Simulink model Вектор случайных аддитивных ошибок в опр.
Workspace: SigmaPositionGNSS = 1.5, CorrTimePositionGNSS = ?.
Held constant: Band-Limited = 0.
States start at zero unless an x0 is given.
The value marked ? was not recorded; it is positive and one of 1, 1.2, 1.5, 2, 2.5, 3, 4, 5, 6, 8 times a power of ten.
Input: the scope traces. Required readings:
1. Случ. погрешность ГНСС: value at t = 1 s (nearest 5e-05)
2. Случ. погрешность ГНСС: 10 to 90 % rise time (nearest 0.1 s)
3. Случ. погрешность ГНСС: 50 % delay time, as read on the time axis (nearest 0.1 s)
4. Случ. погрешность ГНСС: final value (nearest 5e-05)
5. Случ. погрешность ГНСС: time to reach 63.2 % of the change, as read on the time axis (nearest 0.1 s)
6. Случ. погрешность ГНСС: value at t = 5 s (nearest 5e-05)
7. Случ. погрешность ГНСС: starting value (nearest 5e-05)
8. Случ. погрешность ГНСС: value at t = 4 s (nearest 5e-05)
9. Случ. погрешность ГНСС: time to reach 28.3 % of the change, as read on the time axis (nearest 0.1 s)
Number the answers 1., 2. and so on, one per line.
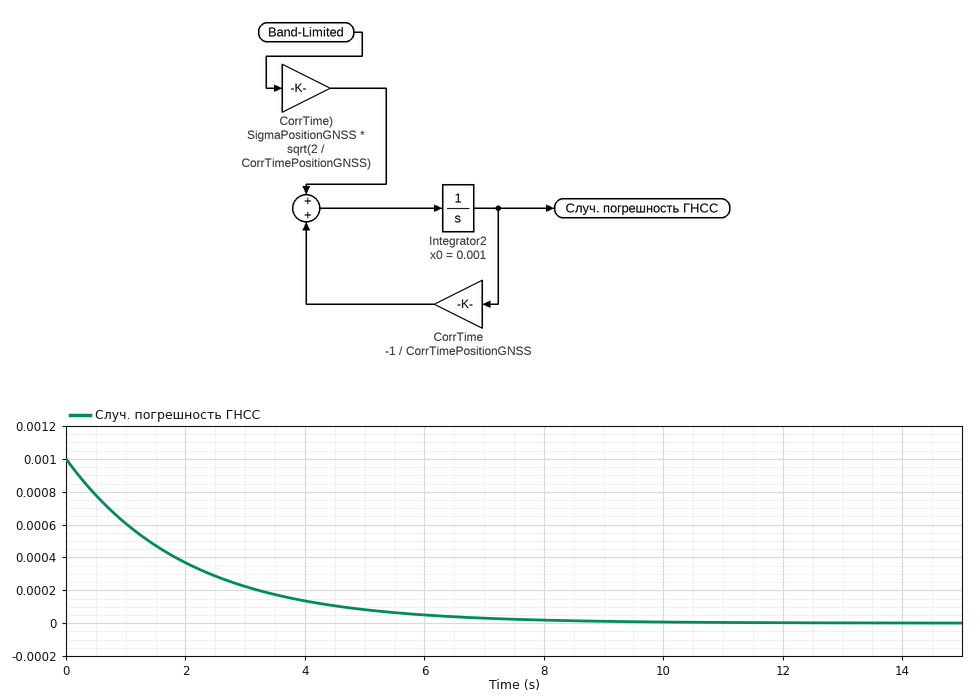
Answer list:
1. 0.00060
2. 4.4 s
3. 1.4 s
4. 0.00000
5. 2.0 s
6. 0.00010
7. 0.00100
8. 0.00015
9. 0.7 s
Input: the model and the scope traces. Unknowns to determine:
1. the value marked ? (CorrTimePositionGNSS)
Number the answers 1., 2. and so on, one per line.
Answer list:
1. 2
